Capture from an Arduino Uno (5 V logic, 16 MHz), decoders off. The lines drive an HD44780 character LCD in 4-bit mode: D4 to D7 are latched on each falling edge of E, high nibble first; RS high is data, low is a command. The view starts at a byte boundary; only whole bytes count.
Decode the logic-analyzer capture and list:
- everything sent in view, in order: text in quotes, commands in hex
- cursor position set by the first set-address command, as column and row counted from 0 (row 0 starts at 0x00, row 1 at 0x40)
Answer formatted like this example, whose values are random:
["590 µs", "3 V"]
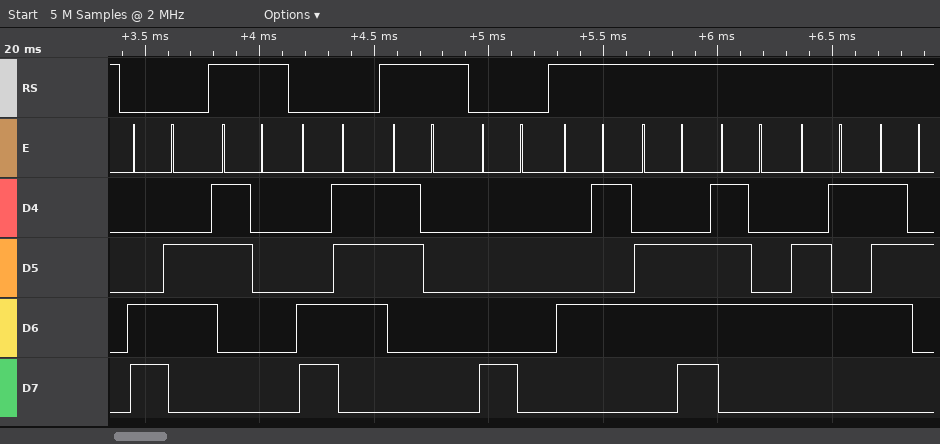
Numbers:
["0xC6 \"0\" 0xC7 \"0\" 0x80 \"Enter\"", "column 6, row 1"]
